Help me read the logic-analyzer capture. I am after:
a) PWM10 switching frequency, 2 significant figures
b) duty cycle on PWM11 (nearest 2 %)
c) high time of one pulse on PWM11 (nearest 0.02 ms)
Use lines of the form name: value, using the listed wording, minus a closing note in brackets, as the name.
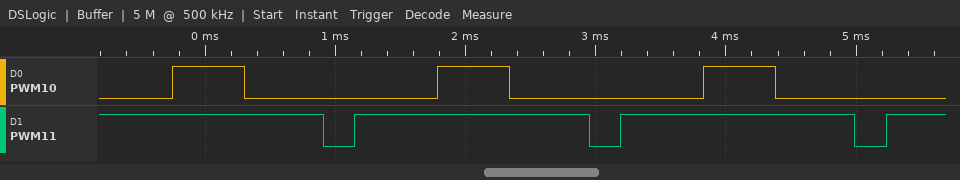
PWM10 switching frequency, 2 significant figures: 490 Hz
duty cycle on PWM11: 88 %
high time of one pulse on PWM11: 1.80 ms
